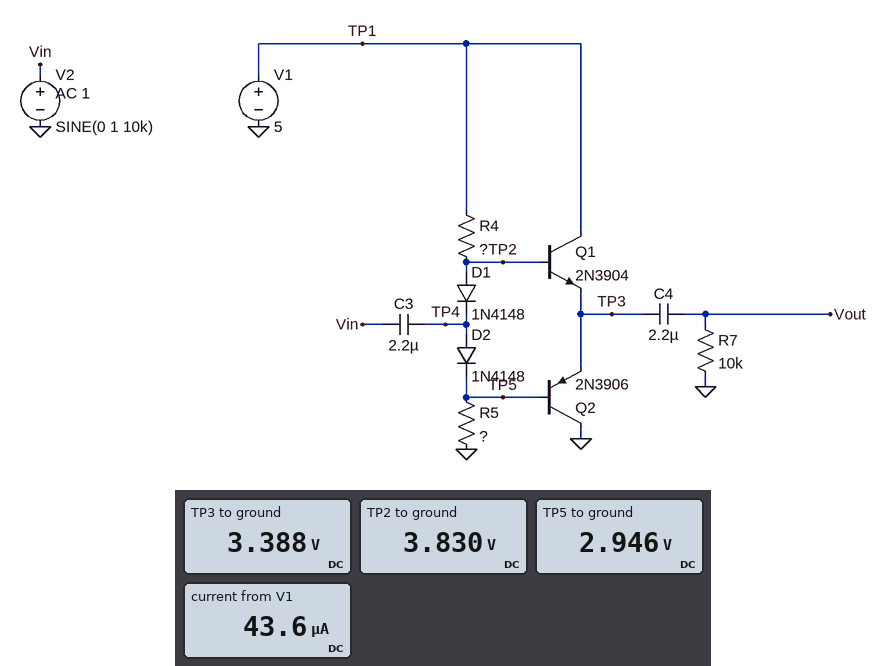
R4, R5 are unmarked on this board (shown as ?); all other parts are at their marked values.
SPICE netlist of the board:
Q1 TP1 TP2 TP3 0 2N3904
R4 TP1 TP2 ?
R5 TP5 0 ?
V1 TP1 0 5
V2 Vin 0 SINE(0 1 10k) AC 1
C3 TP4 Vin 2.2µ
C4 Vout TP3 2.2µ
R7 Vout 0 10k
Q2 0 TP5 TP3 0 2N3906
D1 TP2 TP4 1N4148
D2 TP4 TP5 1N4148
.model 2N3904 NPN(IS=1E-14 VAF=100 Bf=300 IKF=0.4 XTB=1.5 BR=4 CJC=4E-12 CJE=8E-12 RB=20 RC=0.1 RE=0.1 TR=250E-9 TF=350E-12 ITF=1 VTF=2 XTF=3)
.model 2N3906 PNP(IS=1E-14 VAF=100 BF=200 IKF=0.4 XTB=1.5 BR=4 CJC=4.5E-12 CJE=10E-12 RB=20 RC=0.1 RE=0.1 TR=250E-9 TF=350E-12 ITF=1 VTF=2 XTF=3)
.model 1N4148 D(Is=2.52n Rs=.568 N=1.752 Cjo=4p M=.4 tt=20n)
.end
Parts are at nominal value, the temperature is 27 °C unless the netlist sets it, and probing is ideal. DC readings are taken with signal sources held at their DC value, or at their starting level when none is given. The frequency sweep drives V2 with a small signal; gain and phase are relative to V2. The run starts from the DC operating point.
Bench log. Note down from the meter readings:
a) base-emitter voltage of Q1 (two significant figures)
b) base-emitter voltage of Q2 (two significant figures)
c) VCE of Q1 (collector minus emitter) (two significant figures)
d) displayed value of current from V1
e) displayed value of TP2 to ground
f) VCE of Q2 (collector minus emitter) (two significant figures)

440 mV
-440 mV
1.6 V
43.6 µA
3.830 V
-3.4 V
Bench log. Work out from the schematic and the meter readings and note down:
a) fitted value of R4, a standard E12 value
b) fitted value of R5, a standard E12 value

27 kΩ
68 kΩ
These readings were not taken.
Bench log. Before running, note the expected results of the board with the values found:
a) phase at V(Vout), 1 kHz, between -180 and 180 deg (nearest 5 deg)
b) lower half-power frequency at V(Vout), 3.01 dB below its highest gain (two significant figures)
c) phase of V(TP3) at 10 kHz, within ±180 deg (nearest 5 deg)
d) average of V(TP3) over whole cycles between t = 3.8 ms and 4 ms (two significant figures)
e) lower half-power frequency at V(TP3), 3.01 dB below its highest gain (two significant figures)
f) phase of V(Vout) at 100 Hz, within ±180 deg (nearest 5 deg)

0 deg
700 kHz
5 deg
3.4 V
700 kHz
5 deg
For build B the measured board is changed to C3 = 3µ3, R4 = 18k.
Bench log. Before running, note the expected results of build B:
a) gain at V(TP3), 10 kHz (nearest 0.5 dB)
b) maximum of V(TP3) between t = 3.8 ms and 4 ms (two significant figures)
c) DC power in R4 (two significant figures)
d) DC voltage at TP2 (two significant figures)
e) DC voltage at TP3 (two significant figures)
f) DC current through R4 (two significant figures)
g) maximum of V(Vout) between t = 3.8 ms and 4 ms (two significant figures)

-14.5 dB
4.4 V
41 µW
4.1 V
3.7 V
48 µA
700 mV
